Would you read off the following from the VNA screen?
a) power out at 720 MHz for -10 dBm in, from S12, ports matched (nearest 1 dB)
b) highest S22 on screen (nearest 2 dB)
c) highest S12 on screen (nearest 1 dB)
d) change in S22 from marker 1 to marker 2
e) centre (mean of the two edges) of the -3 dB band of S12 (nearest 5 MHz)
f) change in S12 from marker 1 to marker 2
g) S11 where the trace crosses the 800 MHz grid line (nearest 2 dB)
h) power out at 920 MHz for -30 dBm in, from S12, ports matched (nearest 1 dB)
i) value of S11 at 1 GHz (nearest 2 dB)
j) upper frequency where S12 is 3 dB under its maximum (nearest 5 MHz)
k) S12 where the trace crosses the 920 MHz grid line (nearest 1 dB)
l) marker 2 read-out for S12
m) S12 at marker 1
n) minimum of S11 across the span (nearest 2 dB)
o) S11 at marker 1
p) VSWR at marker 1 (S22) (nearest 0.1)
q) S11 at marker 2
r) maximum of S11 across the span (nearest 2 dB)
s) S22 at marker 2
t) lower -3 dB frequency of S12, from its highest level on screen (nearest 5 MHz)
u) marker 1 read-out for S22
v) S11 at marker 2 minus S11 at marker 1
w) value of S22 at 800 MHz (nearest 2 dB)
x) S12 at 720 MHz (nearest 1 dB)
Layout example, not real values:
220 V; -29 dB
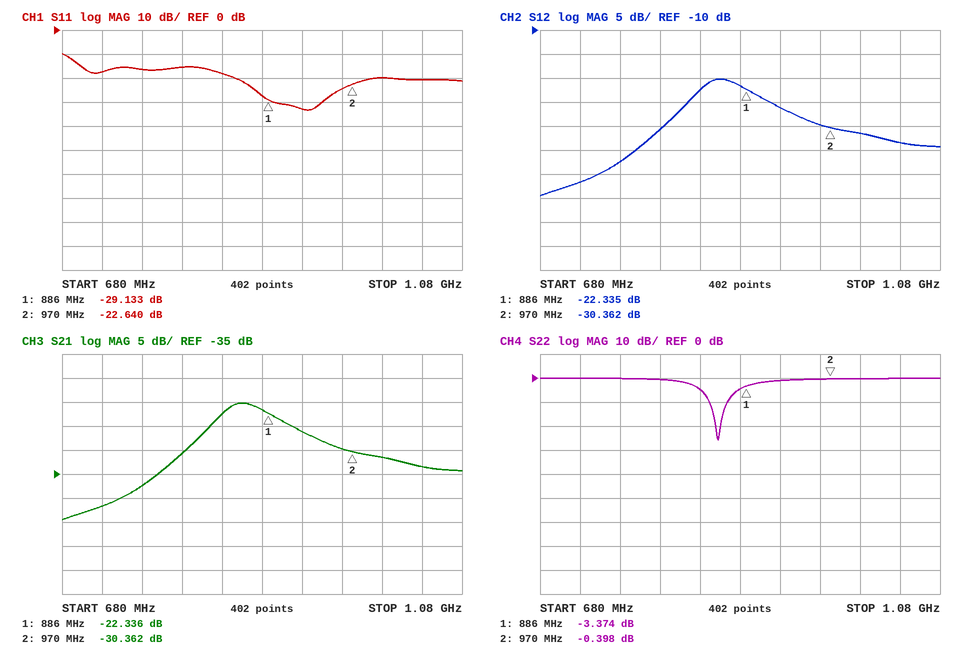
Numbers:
-52 dBm; 0 dB; -20 dB; 2.976 dB; 865 MHz; -8.027 dB; -16 dB; -56 dBm; -20 dB; 895 MHz; -26 dB; -30.362 dB; -22.335 dB; -34 dB; -29.133 dB; 5.2; -22.640 dB; -10 dB; -0.398 dB; 835 MHz; -3.374 dB; 6.493 dB; 0 dB; -42 dB
